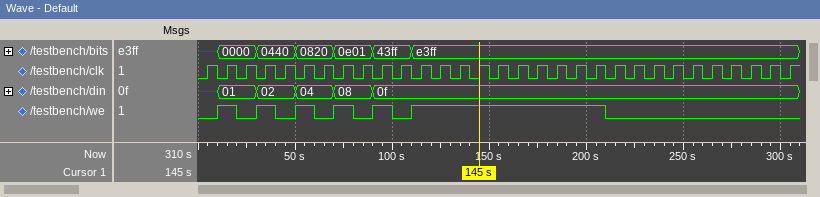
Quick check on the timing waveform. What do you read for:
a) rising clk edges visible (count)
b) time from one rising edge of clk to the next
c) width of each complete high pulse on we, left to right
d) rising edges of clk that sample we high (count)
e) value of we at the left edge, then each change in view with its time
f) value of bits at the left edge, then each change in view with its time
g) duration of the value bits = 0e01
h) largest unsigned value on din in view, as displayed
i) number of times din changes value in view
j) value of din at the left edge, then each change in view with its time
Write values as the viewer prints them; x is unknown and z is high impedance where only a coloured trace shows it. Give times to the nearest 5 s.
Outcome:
31
10 s
10 s, 10 s, 10 s, 10 s, 10 s, 100 s
15
0, 1 at 10 s, 0 at 20 s, 1 at 30 s, 0 at 40 s, 1 at 50 s, 0 at 60 s, 1 at 70 s, 0 at 80 s, 1 at 90 s, 0 at 100 s, 1 at 110 s, 0 at 210 s
x, 0000 at 10 s, 0440 at 30 s, 0820 at 50 s, 0e01 at 70 s, 43ff at 90 s, e3ff at 110 s
20 s
0f
5
x, 01 at 10 s, 02 at 30 s, 04 at 50 s, 08 at 70 s, 0f at 90 s
